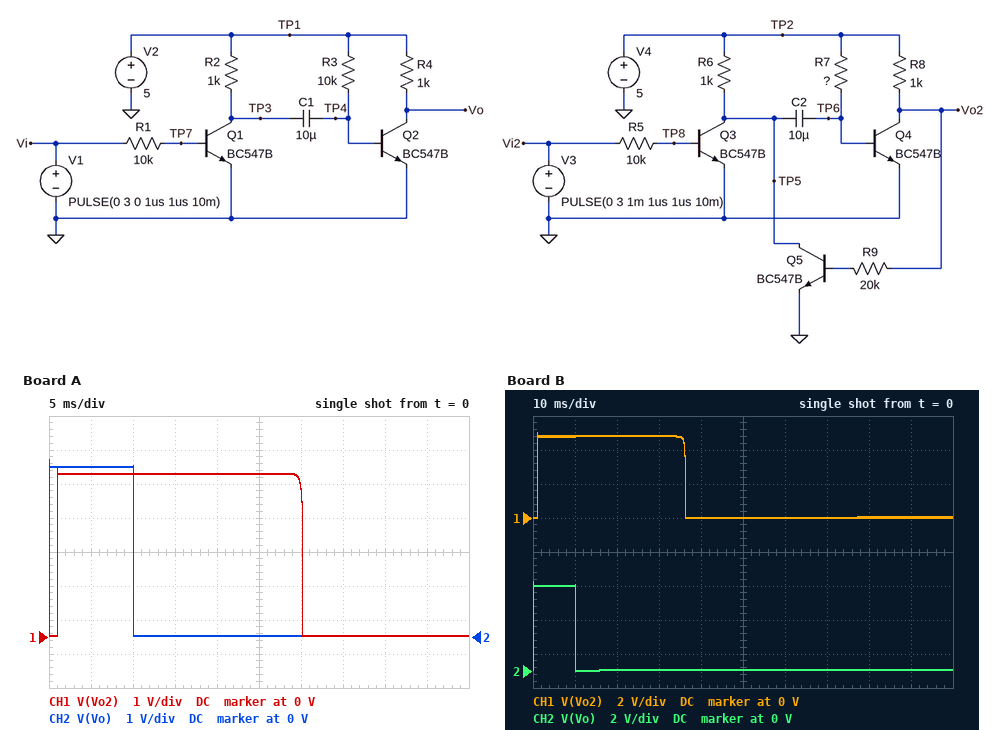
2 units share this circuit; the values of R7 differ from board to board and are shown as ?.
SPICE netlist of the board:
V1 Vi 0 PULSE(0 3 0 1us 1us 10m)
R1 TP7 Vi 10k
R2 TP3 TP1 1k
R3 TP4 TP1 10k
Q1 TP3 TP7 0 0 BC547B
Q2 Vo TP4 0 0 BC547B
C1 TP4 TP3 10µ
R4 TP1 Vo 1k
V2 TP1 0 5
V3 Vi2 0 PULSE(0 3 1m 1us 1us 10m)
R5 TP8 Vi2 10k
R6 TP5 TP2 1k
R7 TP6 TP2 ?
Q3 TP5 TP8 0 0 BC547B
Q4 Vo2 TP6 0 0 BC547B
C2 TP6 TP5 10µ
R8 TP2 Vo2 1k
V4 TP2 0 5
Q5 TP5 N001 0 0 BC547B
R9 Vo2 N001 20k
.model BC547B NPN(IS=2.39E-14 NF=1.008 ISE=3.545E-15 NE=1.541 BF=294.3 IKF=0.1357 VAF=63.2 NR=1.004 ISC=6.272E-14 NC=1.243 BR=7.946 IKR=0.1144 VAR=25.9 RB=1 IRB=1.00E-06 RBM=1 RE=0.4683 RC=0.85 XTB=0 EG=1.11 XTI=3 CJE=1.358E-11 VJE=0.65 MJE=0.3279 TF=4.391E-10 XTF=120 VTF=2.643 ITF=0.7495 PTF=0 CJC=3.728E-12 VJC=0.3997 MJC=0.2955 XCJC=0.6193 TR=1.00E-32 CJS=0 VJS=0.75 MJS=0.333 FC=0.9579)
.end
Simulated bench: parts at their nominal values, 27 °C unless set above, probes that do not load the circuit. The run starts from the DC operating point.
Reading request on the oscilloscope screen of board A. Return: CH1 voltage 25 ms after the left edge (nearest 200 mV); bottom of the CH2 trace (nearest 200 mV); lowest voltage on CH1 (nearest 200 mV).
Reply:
4.8 V
0 V
0 V
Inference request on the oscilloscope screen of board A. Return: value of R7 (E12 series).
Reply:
3.9 kΩ
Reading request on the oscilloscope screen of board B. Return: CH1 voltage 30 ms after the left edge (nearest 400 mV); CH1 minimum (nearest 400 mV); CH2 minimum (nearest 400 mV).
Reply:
4.8 V
0 V
0 V
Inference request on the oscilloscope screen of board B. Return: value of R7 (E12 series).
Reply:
4.7 kΩ
